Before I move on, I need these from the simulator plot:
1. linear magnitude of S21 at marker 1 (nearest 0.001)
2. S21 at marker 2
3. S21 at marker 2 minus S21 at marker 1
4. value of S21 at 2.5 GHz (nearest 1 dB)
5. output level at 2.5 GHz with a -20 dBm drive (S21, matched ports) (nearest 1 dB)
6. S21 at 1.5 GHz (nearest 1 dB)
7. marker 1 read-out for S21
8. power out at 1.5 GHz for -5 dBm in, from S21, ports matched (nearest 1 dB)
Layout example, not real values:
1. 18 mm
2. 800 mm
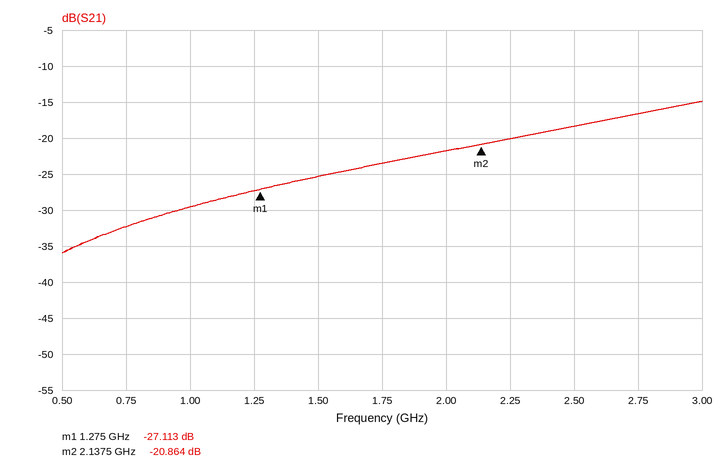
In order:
1. 0.044
2. -20.864 dB
3. 6.249 dB
4. -18 dB
5. -38 dBm
6. -25 dB
7. -27.113 dB
8. -30 dBm
